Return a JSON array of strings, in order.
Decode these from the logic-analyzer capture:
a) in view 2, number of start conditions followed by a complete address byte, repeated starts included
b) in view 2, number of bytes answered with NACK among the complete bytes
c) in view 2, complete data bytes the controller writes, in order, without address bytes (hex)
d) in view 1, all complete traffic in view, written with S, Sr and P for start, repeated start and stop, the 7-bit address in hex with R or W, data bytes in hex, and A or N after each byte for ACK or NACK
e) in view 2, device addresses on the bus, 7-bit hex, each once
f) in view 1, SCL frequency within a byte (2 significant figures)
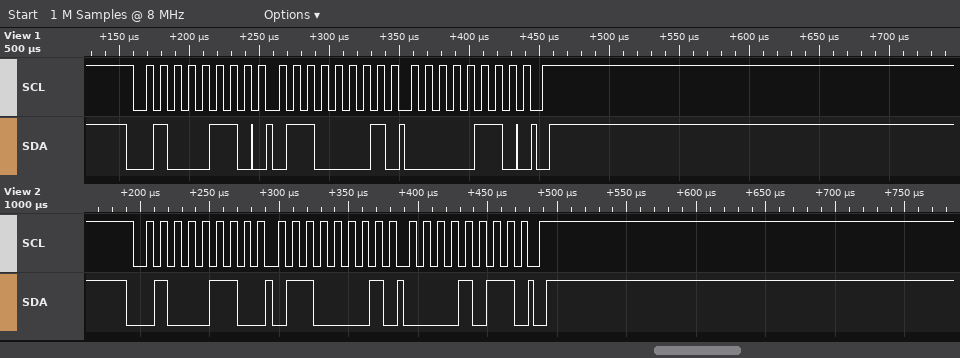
["1", "0", "61 0B", "S 23W A 61 A 06 A P", "0x23", "100 kHz"]
